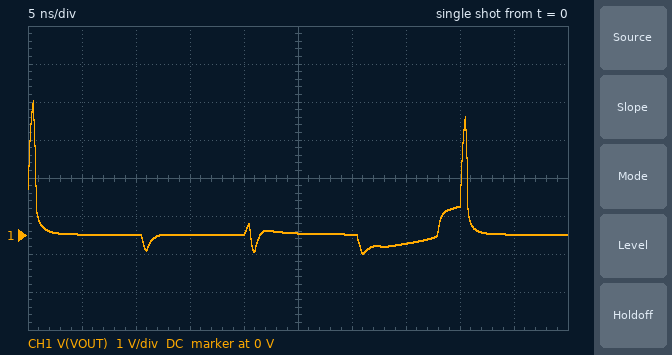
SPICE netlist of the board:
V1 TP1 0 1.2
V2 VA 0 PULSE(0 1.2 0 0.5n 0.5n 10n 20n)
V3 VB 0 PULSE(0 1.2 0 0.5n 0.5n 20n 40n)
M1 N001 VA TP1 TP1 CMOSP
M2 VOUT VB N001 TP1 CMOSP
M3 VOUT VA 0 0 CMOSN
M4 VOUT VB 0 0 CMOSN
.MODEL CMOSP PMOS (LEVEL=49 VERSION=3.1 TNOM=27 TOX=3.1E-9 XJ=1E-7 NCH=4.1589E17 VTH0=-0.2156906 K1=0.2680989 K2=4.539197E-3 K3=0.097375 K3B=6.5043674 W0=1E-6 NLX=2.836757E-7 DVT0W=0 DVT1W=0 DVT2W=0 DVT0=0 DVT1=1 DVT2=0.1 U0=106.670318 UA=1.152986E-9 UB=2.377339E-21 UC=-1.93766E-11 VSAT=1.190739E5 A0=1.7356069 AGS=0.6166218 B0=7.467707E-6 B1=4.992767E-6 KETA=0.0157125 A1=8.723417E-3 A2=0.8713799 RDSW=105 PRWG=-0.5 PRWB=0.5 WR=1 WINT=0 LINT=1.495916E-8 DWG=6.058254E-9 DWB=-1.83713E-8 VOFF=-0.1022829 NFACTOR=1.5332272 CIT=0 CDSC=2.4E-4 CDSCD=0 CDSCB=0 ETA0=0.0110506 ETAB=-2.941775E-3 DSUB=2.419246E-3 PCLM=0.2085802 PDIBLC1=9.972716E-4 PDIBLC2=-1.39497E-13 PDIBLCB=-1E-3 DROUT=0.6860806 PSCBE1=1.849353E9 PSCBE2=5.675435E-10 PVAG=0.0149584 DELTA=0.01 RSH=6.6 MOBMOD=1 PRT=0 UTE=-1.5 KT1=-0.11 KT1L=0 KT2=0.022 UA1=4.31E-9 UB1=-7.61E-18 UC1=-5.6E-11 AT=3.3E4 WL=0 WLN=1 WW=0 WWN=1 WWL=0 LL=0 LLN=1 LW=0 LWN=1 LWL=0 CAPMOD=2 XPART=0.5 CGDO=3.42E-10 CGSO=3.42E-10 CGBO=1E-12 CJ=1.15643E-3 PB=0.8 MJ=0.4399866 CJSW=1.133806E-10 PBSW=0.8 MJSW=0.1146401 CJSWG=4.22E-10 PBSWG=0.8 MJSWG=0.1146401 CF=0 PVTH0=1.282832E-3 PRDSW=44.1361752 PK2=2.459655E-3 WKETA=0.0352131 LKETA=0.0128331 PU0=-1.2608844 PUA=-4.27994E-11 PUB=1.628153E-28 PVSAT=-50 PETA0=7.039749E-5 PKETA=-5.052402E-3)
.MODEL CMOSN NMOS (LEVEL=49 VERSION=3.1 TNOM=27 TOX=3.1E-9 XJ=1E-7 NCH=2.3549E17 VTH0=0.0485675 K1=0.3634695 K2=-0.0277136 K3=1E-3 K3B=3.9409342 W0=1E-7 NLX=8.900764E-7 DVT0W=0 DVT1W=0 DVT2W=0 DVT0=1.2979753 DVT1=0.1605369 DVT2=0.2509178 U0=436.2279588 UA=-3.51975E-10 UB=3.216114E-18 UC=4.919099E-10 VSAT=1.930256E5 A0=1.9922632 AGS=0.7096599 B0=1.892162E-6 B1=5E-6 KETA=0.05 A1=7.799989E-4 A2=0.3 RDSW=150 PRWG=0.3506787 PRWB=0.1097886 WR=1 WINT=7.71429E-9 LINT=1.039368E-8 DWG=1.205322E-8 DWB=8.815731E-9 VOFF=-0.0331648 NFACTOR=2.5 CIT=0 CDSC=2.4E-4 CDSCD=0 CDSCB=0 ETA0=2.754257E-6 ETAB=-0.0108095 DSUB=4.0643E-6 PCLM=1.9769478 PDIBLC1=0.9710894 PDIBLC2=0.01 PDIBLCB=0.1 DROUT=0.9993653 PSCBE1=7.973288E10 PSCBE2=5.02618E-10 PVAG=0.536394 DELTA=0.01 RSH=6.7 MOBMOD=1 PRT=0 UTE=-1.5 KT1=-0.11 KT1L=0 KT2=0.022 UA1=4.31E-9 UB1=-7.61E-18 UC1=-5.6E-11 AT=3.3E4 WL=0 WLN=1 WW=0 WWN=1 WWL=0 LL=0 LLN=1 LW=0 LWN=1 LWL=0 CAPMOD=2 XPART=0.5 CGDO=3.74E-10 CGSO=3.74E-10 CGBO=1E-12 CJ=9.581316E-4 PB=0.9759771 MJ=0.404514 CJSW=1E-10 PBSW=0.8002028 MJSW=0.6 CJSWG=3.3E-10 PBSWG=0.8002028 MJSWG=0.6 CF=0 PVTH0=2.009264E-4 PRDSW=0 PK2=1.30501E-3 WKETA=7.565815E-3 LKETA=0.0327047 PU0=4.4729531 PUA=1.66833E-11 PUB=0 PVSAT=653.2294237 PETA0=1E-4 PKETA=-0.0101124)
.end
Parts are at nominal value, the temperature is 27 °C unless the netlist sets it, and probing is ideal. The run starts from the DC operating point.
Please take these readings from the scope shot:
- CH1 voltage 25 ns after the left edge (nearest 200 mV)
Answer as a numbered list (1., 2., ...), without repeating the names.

1. 0 V
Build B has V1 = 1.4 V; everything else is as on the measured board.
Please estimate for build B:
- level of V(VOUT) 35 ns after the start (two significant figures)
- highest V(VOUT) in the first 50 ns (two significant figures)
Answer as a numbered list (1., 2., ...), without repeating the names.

1. -200 mV
2. 3.7 V
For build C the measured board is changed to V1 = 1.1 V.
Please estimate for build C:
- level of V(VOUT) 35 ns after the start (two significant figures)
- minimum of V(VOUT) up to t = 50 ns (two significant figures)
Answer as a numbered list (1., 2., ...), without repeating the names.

1. -240 mV
2. -510 mV
